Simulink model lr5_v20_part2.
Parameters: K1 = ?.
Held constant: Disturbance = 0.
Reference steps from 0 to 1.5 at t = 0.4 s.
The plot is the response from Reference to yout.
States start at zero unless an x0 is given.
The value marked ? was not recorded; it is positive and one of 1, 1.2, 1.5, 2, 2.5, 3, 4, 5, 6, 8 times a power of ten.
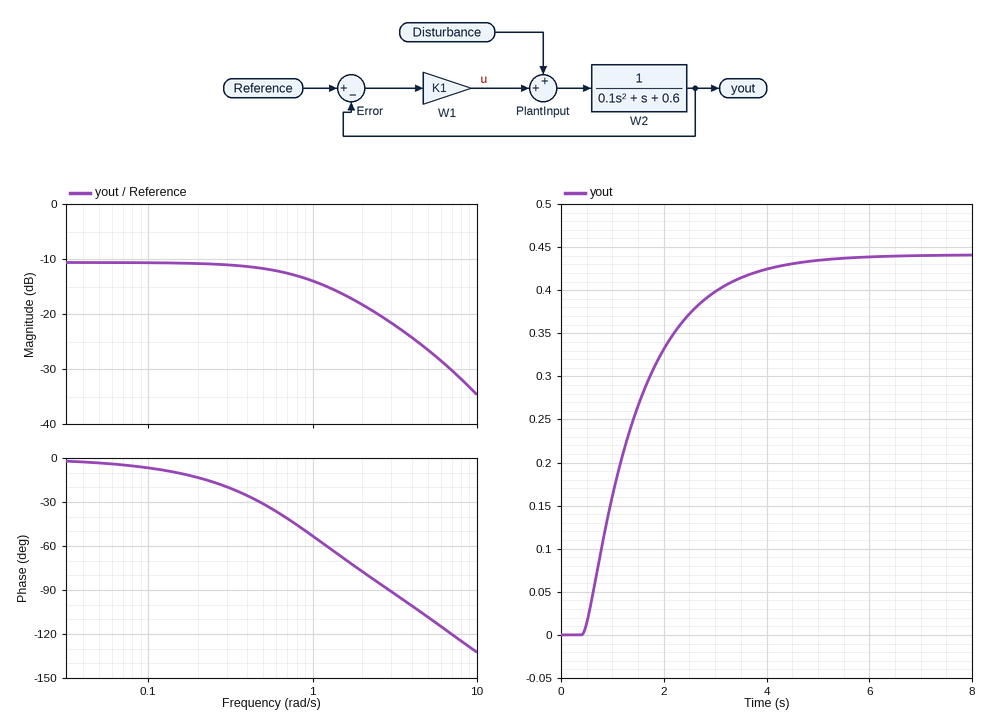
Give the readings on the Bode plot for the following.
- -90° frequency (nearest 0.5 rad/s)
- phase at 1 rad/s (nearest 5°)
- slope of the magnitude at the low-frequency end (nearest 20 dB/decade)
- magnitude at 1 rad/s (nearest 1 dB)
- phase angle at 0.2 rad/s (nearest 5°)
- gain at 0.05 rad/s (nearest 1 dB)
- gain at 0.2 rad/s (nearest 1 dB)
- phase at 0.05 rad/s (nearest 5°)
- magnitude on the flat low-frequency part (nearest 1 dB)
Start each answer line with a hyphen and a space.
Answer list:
- 3.0 rad/s
- -55°
- 0 dB/decade
- -14 dB
- -15°
- -11 dB
- -11 dB
- -5°
- -11 dB
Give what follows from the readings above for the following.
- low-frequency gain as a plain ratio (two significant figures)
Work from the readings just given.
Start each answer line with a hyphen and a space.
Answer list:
- 0.28
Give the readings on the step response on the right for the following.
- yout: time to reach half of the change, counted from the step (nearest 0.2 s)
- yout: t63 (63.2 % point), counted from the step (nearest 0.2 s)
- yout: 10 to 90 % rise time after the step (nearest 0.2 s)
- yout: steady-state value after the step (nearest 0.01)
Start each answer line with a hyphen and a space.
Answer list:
- 0.8 s
- 1.2 s
- 2.4 s
- 0.44
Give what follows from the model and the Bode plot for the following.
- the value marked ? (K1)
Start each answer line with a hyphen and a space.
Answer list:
- 0.25
